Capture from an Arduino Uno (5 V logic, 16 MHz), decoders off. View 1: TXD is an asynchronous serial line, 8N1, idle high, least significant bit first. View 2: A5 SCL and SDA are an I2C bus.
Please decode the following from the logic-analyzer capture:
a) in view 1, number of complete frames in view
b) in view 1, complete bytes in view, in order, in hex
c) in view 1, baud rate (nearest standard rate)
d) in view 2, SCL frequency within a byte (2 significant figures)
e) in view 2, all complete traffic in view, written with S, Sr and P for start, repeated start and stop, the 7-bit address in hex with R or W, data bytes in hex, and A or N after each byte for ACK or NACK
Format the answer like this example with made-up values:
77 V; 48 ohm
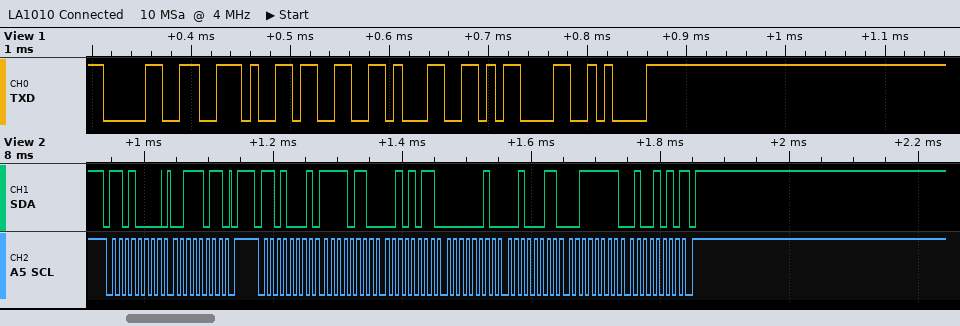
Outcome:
6; 0x30 0x2E 0x33 0x31 0x0D 0x0A; 115200 baud; 100 kHz; S 68W A 3B A P S 68R A F6 A 2B A 02 A 23 A 3F A 4A N P
